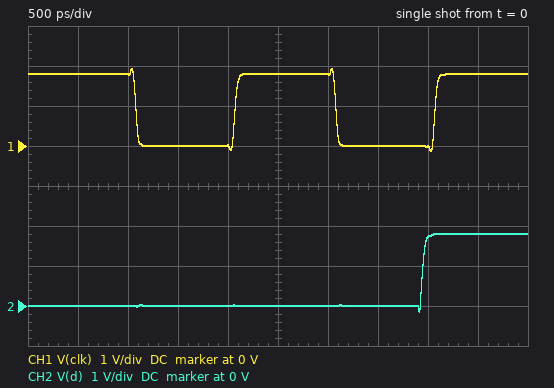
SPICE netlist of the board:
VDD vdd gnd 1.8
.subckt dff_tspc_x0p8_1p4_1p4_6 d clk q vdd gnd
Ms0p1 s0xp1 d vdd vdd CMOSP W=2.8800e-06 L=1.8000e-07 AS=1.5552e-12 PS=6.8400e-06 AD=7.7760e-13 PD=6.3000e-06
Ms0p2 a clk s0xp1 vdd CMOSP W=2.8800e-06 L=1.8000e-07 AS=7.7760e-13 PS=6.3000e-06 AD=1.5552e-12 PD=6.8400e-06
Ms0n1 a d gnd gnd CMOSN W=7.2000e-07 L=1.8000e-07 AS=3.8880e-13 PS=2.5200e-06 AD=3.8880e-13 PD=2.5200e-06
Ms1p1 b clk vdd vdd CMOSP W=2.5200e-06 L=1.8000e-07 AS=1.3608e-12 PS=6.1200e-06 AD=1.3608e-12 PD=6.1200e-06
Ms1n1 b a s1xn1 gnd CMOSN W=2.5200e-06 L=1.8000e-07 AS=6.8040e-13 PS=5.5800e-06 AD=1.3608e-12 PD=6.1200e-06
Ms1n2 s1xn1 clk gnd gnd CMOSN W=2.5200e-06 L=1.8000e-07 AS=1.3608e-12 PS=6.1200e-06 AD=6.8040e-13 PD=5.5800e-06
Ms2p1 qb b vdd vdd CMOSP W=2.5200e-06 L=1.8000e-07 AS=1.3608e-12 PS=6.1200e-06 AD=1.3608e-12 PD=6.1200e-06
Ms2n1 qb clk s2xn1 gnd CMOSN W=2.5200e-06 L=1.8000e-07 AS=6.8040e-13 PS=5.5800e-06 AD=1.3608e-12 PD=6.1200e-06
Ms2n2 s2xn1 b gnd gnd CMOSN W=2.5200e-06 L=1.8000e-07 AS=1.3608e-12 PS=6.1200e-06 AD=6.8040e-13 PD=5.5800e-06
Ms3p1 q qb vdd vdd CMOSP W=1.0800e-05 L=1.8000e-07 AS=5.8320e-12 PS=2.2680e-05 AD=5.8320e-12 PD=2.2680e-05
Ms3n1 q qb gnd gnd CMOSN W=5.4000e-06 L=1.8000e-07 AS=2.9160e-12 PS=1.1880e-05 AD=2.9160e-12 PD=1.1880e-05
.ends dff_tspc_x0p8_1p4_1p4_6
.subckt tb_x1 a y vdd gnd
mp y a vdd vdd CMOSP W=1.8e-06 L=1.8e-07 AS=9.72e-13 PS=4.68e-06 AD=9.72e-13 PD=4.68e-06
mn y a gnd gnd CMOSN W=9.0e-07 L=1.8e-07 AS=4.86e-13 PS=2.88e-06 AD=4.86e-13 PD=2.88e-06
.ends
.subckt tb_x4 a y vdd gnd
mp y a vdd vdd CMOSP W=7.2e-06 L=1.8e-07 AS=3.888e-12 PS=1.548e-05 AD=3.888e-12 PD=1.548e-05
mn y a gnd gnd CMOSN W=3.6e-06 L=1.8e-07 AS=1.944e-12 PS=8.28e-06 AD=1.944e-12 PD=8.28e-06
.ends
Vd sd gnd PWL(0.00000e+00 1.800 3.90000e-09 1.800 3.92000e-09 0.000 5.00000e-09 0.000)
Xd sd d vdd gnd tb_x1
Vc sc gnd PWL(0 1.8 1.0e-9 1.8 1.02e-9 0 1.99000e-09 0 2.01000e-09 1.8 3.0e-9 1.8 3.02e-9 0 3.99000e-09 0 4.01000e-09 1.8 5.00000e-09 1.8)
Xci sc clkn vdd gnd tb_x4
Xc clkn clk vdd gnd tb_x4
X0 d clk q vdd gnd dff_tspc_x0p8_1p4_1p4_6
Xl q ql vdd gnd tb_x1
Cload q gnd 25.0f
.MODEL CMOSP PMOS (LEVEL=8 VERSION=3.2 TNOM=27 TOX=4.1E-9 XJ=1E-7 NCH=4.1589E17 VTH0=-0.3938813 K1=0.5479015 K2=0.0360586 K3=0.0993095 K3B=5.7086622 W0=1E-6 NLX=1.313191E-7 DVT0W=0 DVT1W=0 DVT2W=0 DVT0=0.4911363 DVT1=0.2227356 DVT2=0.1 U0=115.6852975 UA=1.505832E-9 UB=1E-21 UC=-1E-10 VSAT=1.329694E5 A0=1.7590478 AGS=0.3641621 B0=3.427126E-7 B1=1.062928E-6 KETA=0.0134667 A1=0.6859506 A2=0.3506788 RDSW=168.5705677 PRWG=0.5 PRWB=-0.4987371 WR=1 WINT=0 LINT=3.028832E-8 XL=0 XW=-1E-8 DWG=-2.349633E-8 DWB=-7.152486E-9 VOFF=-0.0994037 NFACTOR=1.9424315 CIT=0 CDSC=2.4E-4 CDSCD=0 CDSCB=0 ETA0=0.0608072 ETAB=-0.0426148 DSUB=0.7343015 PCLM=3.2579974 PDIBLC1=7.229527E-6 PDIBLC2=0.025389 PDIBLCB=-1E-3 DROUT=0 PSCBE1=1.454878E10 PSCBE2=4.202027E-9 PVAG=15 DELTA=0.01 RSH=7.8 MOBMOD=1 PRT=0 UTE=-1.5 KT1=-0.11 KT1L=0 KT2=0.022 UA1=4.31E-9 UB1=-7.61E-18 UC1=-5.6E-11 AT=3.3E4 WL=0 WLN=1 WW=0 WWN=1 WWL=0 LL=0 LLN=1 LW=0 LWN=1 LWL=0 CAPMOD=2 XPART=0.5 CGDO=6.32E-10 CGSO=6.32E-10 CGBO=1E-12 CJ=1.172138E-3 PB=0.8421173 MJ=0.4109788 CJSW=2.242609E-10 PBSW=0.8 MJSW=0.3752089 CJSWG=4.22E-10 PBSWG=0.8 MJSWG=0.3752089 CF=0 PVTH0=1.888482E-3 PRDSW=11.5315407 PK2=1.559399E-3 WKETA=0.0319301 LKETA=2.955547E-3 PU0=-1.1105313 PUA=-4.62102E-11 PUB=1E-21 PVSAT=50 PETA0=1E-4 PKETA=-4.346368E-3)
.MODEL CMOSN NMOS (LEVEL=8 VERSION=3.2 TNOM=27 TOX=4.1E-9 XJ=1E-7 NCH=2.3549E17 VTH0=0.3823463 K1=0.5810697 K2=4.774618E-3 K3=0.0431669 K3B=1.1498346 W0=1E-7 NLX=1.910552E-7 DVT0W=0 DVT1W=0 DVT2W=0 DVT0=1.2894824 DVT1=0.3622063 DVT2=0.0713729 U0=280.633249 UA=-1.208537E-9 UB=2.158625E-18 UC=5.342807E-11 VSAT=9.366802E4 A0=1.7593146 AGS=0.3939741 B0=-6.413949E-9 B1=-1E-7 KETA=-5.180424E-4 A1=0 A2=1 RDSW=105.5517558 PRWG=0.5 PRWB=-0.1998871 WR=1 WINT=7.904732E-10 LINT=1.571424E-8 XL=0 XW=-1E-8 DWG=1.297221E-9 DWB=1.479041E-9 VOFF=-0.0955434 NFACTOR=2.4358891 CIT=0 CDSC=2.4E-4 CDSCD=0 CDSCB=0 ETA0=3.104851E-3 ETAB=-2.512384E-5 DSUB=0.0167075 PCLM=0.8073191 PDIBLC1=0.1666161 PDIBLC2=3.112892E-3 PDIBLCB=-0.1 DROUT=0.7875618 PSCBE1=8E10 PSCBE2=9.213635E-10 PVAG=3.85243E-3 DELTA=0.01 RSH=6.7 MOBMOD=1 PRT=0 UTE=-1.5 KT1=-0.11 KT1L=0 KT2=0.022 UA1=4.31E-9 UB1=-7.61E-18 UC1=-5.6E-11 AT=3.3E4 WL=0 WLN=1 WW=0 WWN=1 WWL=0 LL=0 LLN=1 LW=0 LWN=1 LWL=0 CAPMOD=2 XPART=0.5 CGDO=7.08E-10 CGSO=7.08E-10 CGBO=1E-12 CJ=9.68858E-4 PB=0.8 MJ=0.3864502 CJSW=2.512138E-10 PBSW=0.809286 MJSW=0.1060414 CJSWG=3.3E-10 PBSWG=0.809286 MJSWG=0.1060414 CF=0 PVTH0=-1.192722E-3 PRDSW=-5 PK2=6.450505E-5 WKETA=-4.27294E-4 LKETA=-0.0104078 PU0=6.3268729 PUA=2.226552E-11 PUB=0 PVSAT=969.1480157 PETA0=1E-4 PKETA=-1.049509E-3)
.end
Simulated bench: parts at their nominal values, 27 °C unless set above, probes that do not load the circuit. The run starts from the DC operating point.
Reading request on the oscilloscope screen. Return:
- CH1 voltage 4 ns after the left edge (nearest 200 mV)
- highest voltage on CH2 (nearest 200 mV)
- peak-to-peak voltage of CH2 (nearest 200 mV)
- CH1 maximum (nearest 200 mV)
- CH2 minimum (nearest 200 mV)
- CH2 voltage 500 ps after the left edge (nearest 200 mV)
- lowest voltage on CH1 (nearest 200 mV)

0 V
1.8 V
2.0 V
2.0 V
-200 mV
0 V
-200 mV
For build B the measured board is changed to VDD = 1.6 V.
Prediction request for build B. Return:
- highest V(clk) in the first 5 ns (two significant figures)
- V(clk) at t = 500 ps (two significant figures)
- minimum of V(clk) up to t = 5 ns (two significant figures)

1.7 V
1.6 V
-150 mV
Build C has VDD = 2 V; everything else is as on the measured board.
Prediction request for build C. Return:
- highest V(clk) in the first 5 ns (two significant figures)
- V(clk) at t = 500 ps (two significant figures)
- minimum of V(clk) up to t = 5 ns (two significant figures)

2.1 V
2.0 V
-120 mV
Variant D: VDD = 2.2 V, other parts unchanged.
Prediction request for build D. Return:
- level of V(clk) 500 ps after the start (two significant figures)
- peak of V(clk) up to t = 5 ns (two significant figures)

2.2 V
2.3 V
